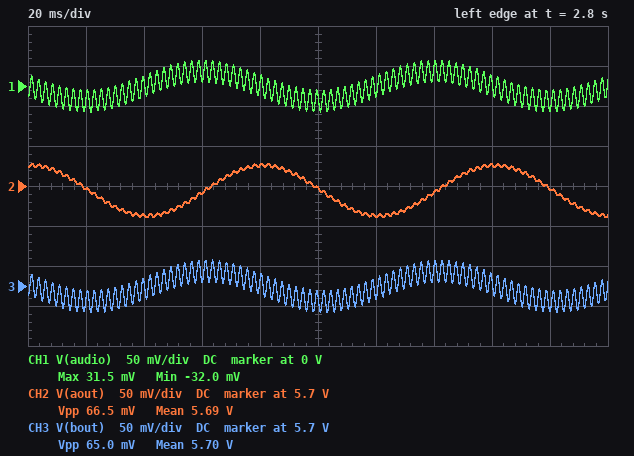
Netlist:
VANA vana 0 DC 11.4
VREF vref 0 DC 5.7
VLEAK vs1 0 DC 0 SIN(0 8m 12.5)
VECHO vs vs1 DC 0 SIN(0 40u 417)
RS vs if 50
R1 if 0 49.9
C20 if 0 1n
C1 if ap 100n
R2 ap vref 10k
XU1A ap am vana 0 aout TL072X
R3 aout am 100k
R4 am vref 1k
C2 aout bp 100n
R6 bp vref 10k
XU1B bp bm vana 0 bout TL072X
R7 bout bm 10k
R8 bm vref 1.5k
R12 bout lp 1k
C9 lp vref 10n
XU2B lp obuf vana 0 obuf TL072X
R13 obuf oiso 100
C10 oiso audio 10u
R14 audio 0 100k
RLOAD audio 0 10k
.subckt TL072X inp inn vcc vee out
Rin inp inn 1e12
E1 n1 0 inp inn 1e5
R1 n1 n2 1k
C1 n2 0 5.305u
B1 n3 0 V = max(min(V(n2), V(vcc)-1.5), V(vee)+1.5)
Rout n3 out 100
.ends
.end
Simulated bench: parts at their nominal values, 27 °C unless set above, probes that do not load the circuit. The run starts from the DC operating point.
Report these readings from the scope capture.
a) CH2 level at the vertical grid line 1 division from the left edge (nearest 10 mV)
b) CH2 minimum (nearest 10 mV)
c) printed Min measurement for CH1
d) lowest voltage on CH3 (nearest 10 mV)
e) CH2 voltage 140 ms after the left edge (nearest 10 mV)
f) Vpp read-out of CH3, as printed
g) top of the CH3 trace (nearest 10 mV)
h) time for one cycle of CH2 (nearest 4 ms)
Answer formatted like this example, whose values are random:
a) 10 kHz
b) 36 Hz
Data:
a) 5.70 V
b) 5.66 V
c) -32.0 mV
d) 5.67 V
e) 5.69 V
f) 65.0 mV
g) 5.73 V
h) 80 ms
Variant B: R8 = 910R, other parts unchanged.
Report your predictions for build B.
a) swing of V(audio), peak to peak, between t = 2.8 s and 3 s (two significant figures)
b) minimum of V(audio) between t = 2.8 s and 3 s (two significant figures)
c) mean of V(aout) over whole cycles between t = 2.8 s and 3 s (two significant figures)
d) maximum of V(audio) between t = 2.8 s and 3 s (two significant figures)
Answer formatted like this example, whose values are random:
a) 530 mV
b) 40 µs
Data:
a) 100 mV
b) -50 mV
c) 5.7 V
d) 50 mV
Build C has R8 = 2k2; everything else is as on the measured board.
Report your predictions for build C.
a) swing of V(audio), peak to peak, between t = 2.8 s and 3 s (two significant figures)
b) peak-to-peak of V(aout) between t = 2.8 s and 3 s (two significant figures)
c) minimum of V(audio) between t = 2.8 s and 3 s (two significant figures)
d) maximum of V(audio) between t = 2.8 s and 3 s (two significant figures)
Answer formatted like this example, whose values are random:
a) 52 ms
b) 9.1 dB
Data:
a) 46 mV
b) 67 mV
c) -23 mV
d) 23 mV
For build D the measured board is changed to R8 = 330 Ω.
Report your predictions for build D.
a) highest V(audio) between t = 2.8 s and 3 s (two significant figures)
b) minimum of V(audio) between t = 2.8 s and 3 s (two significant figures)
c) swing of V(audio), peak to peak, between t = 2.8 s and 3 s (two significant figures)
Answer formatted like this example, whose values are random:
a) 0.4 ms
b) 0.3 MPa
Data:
a) 130 mV
b) -130 mV
c) 260 mV
